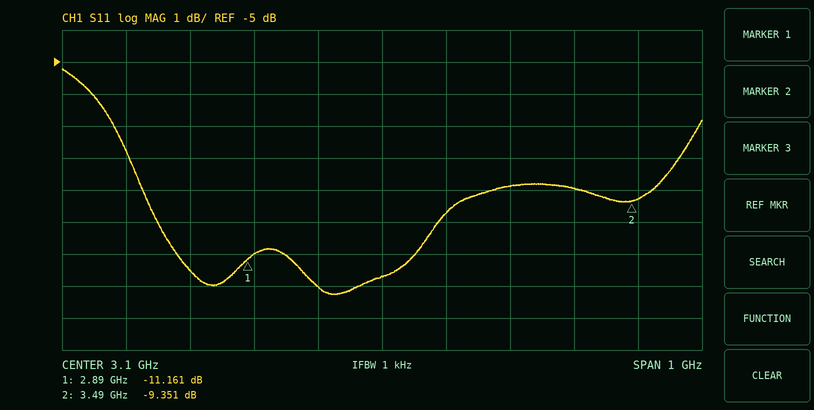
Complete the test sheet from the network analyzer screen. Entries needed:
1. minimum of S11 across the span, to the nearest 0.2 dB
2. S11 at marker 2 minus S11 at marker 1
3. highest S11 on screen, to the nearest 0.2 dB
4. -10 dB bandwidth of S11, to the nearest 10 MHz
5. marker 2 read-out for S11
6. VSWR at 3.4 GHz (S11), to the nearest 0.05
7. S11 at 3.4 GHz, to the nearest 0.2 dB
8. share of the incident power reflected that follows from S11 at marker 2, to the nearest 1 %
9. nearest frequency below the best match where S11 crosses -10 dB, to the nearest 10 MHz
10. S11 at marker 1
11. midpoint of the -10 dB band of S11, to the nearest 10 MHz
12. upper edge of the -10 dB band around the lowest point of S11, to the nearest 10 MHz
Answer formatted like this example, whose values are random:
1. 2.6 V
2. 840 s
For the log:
1. -12.2 dB
2. 1.810 dB
3. -5.2 dB
4. 440 MHz
5. -9.351 dB
6. 2.10
7. -9.0 dB
8. 12 %
9. 2.75 GHz
10. -11.161 dB
11. 2.97 GHz
12. 3.19 GHz
